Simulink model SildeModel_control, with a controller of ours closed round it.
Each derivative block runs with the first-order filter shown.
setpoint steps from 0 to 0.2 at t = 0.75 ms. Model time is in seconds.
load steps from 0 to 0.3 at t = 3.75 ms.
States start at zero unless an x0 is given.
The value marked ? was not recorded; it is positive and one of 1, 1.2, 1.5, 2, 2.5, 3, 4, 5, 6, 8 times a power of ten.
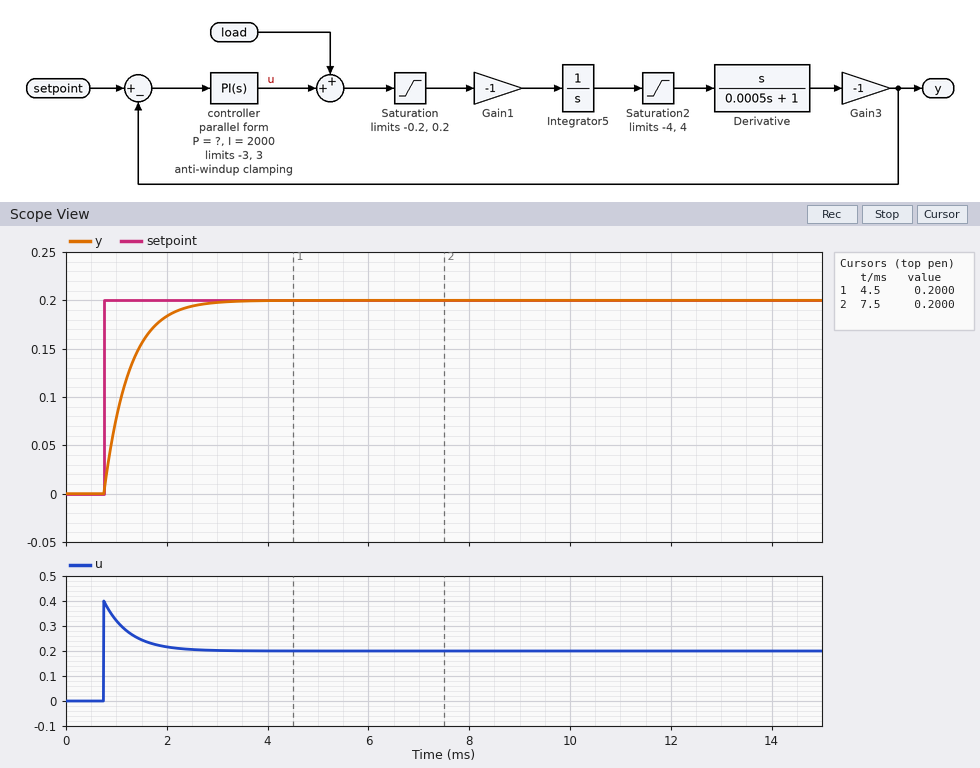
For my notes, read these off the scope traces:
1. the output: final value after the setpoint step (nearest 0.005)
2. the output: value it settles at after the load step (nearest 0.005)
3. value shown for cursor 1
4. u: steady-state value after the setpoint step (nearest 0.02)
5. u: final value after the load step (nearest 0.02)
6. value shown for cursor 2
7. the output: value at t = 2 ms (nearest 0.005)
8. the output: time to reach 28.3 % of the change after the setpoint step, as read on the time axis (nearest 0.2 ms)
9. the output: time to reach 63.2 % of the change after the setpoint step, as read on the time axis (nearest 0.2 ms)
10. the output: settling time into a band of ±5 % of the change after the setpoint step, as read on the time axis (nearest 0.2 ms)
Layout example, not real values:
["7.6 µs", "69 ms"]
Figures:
["0.200", "0.200", "0.2000", "0.20", "0.20", "0.2000", "0.185", "1.0 ms", "1.2 ms", "2.2 ms"]
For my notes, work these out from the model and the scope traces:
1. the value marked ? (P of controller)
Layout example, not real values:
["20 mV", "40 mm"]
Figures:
["2"]
